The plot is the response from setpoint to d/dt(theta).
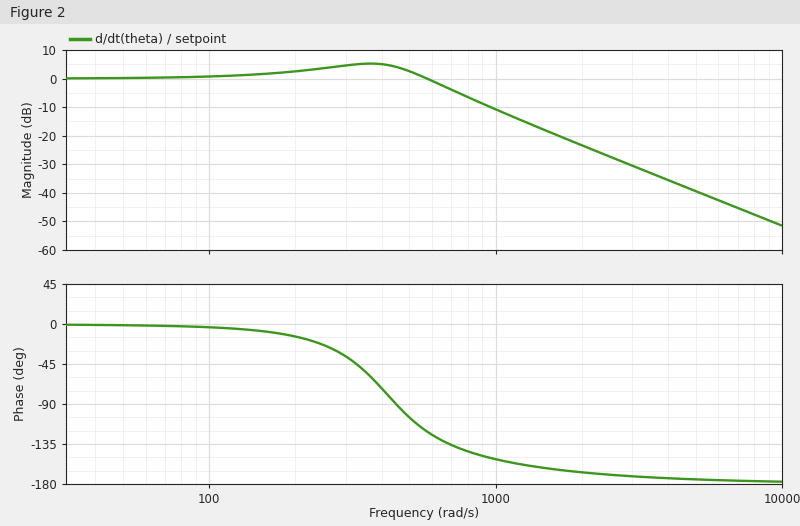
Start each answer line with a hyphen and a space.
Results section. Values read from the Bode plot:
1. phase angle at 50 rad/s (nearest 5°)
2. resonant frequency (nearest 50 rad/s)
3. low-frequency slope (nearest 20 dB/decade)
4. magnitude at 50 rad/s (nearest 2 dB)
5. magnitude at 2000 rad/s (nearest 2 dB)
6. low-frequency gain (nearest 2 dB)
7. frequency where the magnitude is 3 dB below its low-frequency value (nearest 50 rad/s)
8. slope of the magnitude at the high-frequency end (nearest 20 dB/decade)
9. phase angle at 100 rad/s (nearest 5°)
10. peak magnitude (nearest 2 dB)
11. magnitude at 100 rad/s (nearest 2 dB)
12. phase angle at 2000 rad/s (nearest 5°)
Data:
- 0°
- 350 rad/s
- 0 dB/decade
- 0 dB
- -24 dB
- 0 dB
- 650 rad/s
- -40 dB/decade
- -5°
- 6 dB
- 0 dB
- -165°
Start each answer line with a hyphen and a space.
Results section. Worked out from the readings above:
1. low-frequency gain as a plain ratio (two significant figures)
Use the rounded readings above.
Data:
- 1.0
